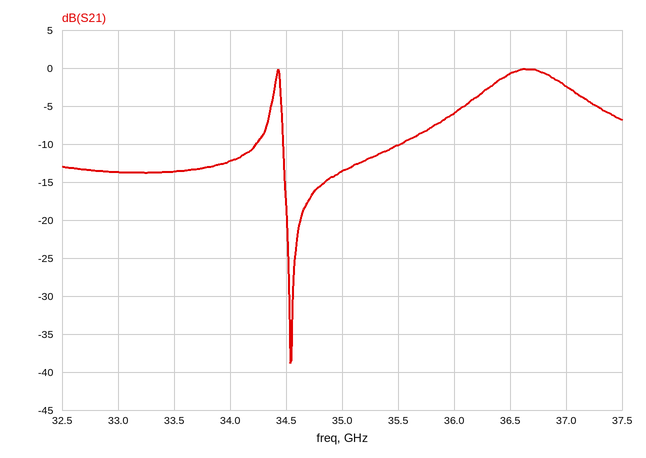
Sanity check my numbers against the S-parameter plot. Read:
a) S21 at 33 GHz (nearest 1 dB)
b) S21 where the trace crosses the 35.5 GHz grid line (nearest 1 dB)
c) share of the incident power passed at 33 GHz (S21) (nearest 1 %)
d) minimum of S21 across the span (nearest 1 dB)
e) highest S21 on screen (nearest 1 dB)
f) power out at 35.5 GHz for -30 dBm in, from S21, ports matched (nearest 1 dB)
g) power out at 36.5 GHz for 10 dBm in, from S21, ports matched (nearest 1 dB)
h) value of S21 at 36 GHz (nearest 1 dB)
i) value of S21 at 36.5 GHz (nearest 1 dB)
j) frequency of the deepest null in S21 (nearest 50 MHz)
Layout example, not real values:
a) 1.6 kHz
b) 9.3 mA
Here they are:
a) -14 dB
b) -10 dB
c) 4 %
d) -39 dB
e) 0 dB
f) -40 dBm
g) 9 dBm
h) -6 dB
i) -1 dB
j) 34.55 GHz
